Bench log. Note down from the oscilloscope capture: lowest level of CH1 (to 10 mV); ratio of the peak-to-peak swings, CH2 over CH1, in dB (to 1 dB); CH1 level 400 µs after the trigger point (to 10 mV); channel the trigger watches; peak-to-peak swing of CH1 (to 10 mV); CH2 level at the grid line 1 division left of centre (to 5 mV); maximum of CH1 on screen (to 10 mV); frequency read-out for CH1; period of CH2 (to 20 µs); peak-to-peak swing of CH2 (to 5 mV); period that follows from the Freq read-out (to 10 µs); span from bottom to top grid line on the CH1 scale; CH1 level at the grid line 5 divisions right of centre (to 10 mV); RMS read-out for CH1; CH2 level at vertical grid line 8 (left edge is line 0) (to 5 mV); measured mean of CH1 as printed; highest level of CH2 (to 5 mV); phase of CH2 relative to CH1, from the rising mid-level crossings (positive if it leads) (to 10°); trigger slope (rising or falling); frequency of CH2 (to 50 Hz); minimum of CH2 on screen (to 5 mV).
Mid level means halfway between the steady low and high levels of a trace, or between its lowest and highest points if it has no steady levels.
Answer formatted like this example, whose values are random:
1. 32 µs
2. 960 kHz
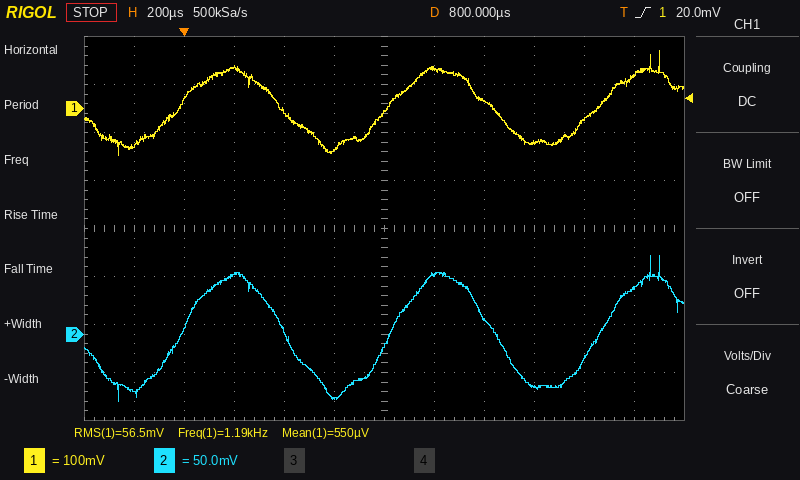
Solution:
1. -100 mV
2. -3 dB
3. -10 mV
4. CH1
5. 220 mV
6. -65 mV
7. 120 mV
8. 1.19 kHz
9. 840 µs
10. 150 mV
11. 840 µs
12. 800 mV
13. 70 mV
14. 56.5 mV
15. 15 mV
16. 550 µV
17. 80 mV
18. 0°
19. rising
20. 1.20 kHz
21. -70 mV
